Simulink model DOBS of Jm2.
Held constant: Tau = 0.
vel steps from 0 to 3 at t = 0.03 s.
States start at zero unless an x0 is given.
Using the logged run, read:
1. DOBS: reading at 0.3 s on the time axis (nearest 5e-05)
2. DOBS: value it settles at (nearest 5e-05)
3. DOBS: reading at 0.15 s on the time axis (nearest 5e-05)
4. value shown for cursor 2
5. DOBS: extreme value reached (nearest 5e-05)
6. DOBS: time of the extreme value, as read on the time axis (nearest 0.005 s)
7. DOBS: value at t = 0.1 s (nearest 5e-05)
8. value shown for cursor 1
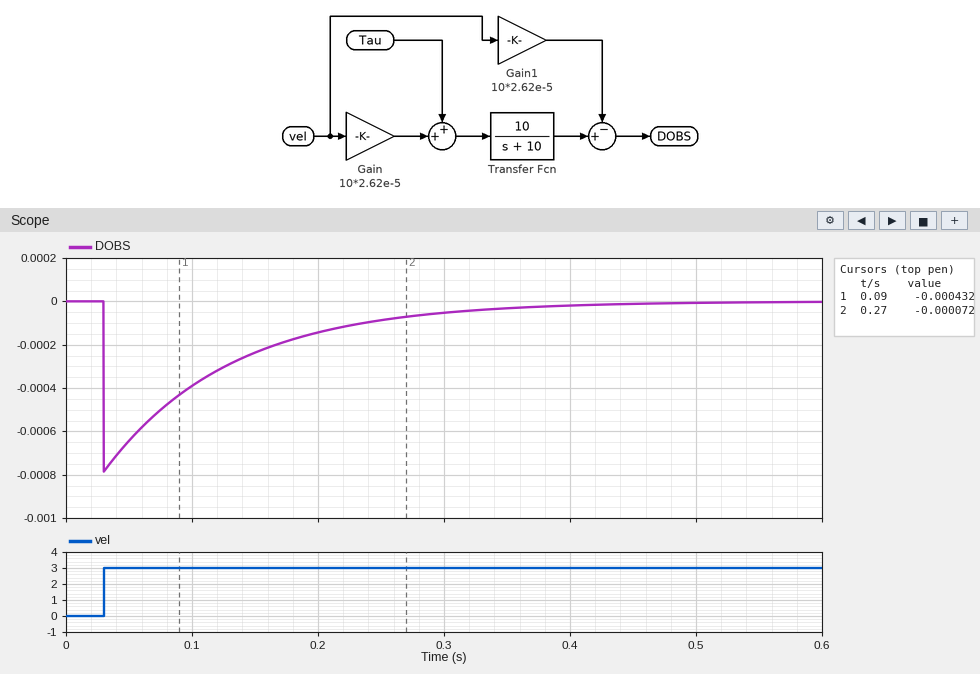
-0.00005
0.00000
-0.00025
-0.000072
-0.00080
0.030 s
-0.00040
-0.000432
